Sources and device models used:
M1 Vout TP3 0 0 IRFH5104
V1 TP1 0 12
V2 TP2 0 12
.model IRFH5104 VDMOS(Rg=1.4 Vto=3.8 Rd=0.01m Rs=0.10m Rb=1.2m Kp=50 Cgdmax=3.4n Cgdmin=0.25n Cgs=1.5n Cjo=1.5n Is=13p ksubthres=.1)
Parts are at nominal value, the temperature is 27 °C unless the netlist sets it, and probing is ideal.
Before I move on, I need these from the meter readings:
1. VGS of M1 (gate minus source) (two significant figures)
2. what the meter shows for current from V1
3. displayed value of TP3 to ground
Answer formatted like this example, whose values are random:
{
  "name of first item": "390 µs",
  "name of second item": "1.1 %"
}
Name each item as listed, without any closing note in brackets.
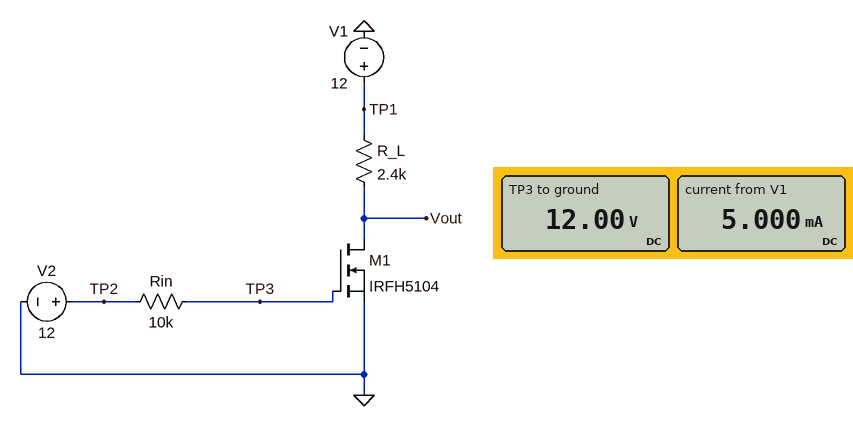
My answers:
{
  "VGS of M1 (gate minus source)": "12 V",
  "what the meter shows for current from V1": "5.000 mA",
  "displayed value of TP3 to ground": "12.00 V"
}
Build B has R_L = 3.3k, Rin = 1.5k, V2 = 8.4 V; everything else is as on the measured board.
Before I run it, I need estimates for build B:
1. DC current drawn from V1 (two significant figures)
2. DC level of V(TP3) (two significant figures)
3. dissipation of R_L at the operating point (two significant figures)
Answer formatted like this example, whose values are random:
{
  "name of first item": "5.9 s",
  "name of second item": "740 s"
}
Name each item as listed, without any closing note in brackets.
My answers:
{
  "DC current drawn from V1": "3.6 mA",
  "DC level of V(TP3)": "8.4 V",
  "dissipation of R_L at the operating point": "44 mW"
}
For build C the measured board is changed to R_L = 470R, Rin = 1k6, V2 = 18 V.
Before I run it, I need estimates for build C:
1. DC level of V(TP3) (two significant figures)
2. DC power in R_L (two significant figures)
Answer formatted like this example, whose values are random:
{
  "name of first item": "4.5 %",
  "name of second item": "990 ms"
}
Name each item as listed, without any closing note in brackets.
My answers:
{
  "DC level of V(TP3)": "18 V",
  "DC power in R_L": "310 mW"
}
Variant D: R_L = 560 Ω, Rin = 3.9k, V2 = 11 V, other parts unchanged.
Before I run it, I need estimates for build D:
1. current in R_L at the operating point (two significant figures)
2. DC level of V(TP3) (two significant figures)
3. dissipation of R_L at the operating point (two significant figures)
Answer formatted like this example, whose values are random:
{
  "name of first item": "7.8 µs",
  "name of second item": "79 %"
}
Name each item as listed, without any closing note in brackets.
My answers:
{
  "current in R_L at the operating point": "21 mA",
  "DC level of V(TP3)": "11 V",
  "dissipation of R_L at the operating point": "260 mW"
}
